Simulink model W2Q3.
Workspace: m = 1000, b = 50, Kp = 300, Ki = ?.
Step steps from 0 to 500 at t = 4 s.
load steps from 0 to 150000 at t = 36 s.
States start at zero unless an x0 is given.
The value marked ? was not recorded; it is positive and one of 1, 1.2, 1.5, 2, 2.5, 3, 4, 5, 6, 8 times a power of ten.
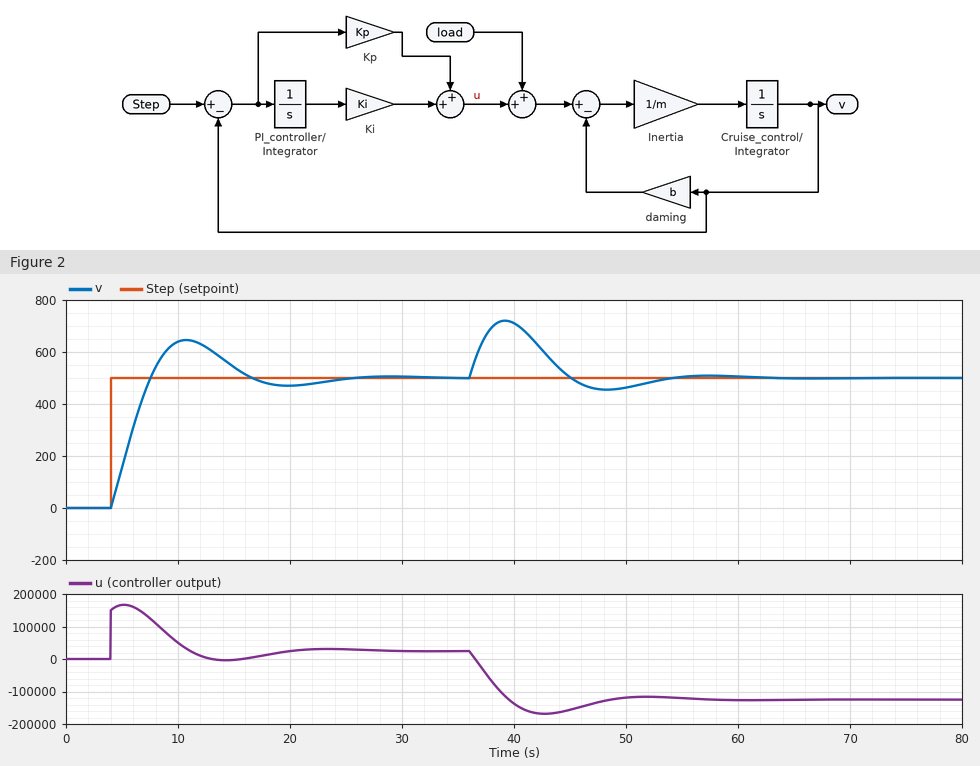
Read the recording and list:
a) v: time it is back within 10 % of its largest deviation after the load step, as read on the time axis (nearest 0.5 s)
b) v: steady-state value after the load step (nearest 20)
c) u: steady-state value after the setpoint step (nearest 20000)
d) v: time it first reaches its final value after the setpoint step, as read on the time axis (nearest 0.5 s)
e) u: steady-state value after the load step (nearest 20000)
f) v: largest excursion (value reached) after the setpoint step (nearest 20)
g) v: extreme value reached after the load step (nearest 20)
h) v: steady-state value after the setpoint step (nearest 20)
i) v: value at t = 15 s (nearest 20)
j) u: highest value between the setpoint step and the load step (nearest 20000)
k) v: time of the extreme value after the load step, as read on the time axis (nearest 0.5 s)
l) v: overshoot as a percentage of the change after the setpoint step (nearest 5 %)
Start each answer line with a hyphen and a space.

- 51.5 s
- 500
- 20000
- 7.5 s
- -120000
- 640
- 720
- 500
- 540
- 160000
- 39.0 s
- 30 %
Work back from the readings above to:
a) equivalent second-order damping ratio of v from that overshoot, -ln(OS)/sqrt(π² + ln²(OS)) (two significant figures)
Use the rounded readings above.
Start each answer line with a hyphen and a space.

- 0.36
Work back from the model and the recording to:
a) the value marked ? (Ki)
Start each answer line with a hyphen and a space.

- 150
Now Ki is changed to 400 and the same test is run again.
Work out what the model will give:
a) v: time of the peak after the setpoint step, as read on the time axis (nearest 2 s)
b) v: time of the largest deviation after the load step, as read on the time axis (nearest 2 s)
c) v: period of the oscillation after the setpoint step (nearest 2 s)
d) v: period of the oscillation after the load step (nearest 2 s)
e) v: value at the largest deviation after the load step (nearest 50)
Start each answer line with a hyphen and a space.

- 8 s
- 38 s
- 10 s
- 10 s
- 650
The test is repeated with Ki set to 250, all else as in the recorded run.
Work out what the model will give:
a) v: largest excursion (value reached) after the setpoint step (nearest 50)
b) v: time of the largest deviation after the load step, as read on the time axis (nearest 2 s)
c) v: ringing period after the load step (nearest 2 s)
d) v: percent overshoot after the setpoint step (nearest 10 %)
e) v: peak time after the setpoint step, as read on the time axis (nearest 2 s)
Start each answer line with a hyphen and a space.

- 700
- 38 s
- 14 s
- 40 %
- 10 s
